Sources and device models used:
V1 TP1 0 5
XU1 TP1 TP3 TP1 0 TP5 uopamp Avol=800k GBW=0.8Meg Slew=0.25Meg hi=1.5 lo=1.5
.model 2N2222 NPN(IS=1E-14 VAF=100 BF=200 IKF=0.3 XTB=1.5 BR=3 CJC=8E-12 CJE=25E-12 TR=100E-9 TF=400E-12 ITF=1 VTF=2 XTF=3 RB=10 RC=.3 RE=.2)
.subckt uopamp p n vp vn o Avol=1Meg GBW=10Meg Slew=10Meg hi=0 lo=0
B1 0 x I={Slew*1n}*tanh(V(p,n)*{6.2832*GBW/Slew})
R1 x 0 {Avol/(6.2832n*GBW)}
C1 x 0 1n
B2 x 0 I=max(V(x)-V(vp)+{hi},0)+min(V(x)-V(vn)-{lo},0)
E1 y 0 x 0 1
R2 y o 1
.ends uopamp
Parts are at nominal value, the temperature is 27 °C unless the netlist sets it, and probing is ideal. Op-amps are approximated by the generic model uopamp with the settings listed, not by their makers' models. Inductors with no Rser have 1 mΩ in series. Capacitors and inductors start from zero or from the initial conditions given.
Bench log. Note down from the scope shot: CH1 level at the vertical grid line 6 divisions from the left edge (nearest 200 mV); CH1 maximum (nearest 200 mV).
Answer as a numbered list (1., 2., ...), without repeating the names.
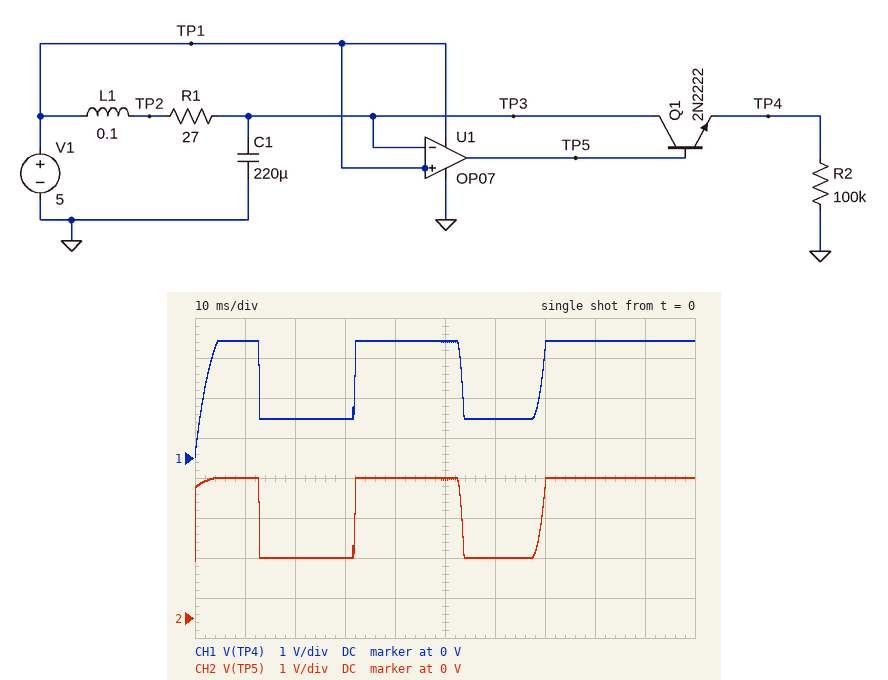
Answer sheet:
1. 1.0 V
2. 3.0 V
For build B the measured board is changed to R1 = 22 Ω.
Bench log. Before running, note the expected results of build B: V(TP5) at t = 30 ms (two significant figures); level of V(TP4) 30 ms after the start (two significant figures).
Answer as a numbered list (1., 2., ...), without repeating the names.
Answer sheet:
1. 3.5 V
2. 2.9 V
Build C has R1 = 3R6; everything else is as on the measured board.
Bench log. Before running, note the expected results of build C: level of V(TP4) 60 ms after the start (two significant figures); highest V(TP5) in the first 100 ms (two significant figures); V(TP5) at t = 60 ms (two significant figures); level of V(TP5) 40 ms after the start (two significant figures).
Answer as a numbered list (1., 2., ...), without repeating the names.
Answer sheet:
1. 2.9 V
2. 3.5 V
3. 3.5 V
4. 1.5 V
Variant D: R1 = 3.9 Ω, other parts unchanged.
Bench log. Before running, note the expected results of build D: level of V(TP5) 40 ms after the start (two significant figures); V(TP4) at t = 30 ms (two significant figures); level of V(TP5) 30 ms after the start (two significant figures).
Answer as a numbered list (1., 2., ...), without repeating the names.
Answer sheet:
1. 1.5 V
2. 2.9 V
3. 3.5 V
